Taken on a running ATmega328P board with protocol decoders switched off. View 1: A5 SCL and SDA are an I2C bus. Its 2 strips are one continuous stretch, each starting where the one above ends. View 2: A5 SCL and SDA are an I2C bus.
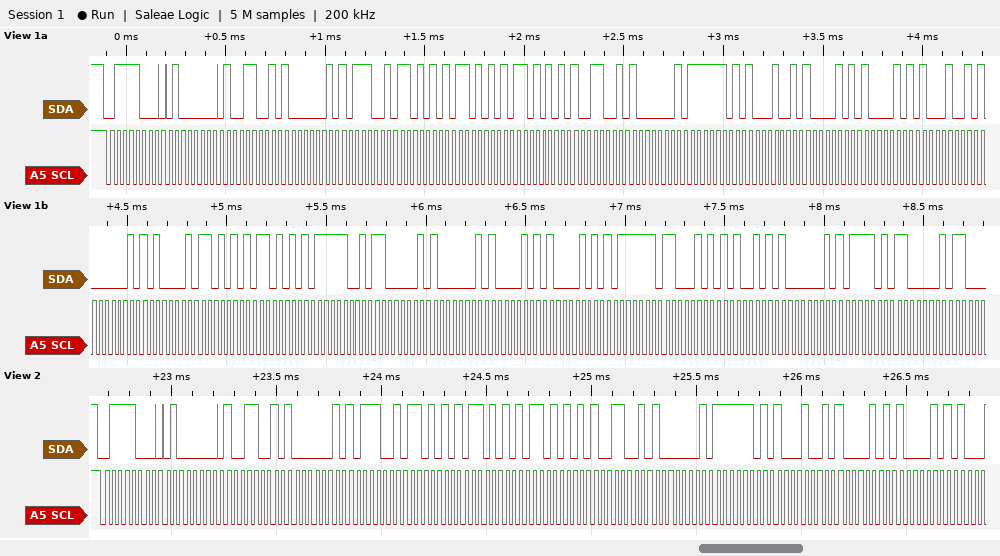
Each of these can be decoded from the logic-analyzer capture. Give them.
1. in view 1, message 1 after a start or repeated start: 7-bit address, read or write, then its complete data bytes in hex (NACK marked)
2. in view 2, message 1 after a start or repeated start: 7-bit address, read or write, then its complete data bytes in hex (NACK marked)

0x3C write: 40 99 81 B9 D5 D5 D5 99 81 FD 89 85 85 89 81 A1 D5 D5 F9 C1 81 85 85 BF C5 A5 81 BD C1
0x3C write: 40 99 81 B9 D5 D5 D5 99 81 FD 89 85 85
